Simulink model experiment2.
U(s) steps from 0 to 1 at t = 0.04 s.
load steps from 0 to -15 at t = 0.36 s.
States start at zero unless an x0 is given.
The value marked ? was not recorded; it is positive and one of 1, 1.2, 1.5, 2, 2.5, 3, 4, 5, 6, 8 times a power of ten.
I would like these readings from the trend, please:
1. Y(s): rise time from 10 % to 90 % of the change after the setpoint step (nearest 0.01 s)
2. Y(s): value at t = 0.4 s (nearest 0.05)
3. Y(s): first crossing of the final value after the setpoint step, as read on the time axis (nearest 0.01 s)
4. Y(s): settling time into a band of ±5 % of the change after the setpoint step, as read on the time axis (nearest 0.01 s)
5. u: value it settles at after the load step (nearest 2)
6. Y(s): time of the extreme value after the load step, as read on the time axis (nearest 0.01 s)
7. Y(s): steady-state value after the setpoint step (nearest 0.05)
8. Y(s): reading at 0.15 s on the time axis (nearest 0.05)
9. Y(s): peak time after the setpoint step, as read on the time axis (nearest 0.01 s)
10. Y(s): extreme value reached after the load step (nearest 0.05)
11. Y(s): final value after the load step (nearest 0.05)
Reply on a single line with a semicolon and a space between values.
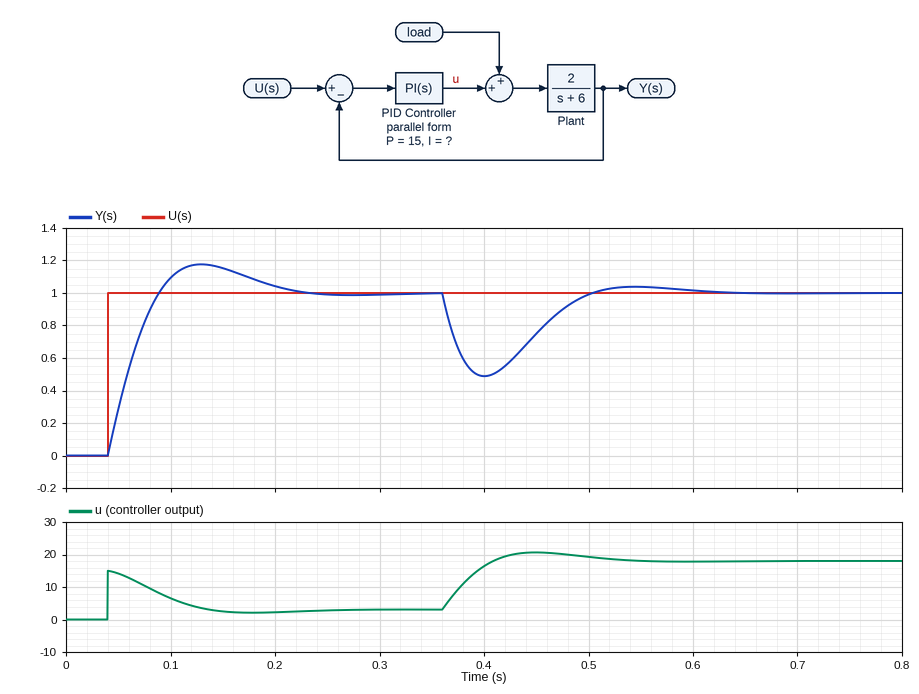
0.04 s; 0.50; 0.09 s; 0.20 s; 18; 0.40 s; 1.00; 1.15; 0.13 s; 0.50; 1.00
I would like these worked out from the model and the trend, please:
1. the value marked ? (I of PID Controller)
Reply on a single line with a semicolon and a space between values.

400
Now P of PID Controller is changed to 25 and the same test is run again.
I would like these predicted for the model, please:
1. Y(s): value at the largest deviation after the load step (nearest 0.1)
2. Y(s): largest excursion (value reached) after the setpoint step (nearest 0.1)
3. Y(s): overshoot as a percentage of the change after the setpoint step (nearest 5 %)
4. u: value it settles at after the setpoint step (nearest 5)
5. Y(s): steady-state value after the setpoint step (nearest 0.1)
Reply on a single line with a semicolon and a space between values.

0.6; 1.1; 10 %; 5; 1.0
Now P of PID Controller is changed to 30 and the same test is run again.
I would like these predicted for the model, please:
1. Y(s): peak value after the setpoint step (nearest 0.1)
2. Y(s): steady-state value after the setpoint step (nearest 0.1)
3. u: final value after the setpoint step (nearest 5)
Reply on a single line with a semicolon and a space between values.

1.1; 1.0; 5
